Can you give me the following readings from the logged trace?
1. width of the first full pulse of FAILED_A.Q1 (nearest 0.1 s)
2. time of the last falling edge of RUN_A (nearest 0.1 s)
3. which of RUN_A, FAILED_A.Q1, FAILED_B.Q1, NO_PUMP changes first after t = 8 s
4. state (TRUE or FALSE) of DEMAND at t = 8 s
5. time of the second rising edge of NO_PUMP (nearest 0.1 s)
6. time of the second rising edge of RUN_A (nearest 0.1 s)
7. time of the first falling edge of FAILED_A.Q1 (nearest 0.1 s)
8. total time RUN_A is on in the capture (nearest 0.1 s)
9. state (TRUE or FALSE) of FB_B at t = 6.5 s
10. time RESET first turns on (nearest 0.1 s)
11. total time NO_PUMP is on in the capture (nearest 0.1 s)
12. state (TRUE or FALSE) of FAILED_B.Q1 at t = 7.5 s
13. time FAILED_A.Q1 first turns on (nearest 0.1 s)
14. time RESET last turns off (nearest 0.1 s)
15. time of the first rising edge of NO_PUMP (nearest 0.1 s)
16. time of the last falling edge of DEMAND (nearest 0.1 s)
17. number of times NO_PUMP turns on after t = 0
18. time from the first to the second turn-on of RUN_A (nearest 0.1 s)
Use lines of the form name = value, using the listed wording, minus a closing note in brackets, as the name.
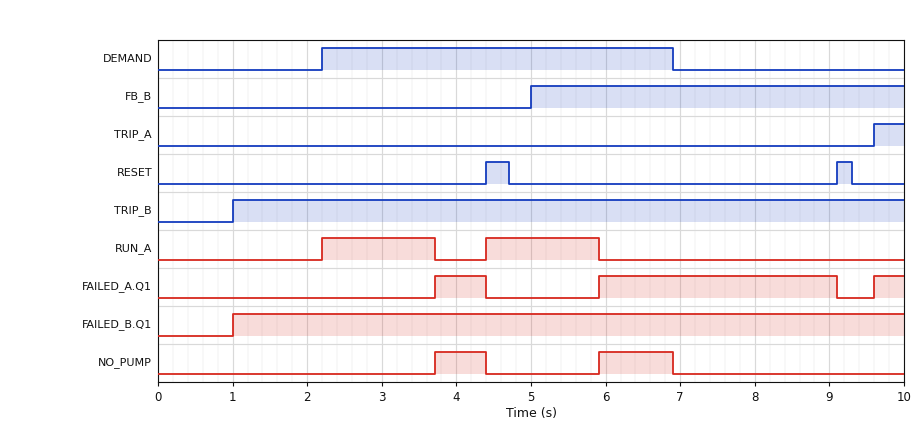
width of the first full pulse of FAILED_A.Q1 = 0.7 s
time of the last falling edge of RUN_A = 5.9 s
which of RUN_A, FAILED_A.Q1, FAILED_B.Q1, NO_PUMP changes first after t = 8 s = FAILED_A.Q1
state (TRUE or FALSE) of DEMAND at t = 8 s = FALSE
time of the second rising edge of NO_PUMP = 5.9 s
time of the second rising edge of RUN_A = 4.4 s
time of the first falling edge of FAILED_A.Q1 = 4.4 s
total time RUN_A is on in the capture = 3.0 s
state (TRUE or FALSE) of FB_B at t = 6.5 s = TRUE
time RESET first turns on = 4.4 s
total time NO_PUMP is on in the capture = 1.7 s
state (TRUE or FALSE) of FAILED_B.Q1 at t = 7.5 s = TRUE
time FAILED_A.Q1 first turns on = 3.7 s
time RESET last turns off = 9.3 s
time of the first rising edge of NO_PUMP = 3.7 s
time of the last falling edge of DEMAND = 6.9 s
number of times NO_PUMP turns on after t = 0 = 2
time from the first to the second turn-on of RUN_A = 2.2 s
